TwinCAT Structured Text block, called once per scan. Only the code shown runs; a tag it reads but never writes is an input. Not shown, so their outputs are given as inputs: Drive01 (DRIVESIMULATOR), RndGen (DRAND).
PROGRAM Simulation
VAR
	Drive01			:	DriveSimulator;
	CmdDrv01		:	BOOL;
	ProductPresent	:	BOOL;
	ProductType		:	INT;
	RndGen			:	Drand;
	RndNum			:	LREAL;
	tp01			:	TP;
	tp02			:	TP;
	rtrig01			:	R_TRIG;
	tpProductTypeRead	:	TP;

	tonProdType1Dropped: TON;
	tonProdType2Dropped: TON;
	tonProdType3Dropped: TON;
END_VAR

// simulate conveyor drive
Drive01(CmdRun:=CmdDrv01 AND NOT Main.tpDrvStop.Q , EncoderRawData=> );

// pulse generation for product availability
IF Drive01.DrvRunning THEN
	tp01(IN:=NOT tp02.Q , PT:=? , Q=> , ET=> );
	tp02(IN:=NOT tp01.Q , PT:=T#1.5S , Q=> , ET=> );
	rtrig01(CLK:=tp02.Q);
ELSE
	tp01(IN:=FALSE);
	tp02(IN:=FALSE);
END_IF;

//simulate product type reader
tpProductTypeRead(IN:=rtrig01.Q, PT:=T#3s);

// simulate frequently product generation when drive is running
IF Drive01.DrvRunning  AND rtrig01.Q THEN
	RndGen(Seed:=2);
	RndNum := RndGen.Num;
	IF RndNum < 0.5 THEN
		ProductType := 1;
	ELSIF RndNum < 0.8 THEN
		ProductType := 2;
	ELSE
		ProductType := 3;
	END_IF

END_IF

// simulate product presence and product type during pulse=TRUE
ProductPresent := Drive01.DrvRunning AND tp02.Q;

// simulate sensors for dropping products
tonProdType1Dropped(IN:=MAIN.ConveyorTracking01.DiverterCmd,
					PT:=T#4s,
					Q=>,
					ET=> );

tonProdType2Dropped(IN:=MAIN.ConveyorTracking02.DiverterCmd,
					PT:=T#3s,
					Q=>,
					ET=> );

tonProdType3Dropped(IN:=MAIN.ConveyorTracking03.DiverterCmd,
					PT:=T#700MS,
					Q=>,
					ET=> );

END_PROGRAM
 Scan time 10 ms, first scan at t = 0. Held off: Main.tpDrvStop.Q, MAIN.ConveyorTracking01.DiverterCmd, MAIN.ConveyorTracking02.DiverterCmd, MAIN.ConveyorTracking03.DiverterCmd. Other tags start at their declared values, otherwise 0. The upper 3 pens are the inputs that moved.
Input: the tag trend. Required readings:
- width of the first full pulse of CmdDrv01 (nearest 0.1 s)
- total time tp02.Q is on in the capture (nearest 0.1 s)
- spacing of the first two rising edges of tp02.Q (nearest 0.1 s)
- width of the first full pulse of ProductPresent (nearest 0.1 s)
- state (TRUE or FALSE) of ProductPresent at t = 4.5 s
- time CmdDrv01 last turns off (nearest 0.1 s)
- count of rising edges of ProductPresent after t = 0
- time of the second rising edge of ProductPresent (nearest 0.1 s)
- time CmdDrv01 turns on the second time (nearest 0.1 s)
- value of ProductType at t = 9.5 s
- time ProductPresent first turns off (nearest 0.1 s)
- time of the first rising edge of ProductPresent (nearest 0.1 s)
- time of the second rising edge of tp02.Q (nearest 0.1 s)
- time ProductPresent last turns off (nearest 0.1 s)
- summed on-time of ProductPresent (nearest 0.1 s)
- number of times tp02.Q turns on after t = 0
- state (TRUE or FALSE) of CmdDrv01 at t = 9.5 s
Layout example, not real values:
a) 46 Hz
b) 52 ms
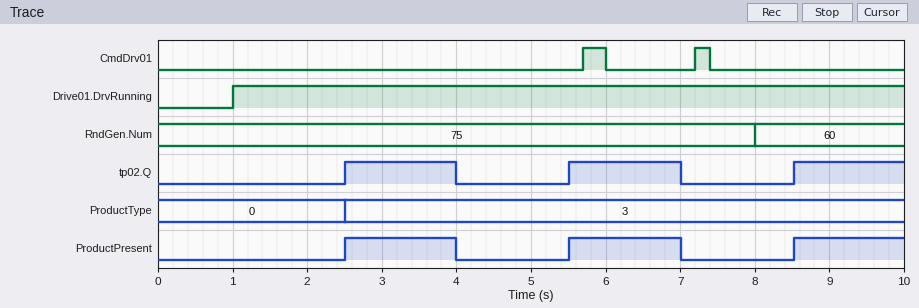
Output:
a) 0.3 s
b) 4.5 s
c) 3.0 s
d) 1.5 s
e) FALSE
f) 7.4 s
g) 3
h) 5.5 s
i) 7.2 s
j) 3
k) 4.0 s
l) 2.5 s
m) 5.5 s
n) 7.0 s
o) 4.5 s
p) 3
q) FALSE
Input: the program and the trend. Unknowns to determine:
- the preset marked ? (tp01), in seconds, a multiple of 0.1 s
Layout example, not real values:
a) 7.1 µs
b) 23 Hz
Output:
a) 1.5 s
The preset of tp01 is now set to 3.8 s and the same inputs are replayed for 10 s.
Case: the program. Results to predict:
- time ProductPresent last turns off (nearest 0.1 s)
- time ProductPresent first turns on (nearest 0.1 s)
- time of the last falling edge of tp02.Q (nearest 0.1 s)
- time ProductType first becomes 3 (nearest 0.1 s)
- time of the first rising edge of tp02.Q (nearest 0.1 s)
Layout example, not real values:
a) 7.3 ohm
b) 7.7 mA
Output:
a) 6.3 s
b) 4.8 s
c) 6.3 s
d) 4.8 s
e) 4.8 s
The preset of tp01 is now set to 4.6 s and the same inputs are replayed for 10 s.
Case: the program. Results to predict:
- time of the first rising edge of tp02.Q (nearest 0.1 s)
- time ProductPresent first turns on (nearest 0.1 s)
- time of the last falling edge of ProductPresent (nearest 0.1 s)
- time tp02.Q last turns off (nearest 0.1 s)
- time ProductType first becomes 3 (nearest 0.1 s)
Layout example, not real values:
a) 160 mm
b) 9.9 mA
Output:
a) 5.6 s
b) 5.6 s
c) 7.1 s
d) 7.1 s
e) 5.6 s
